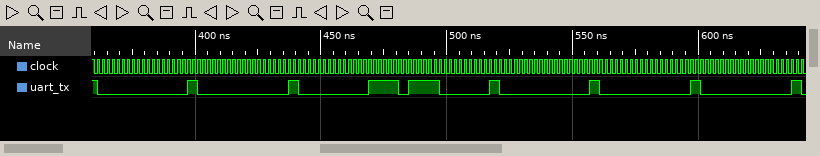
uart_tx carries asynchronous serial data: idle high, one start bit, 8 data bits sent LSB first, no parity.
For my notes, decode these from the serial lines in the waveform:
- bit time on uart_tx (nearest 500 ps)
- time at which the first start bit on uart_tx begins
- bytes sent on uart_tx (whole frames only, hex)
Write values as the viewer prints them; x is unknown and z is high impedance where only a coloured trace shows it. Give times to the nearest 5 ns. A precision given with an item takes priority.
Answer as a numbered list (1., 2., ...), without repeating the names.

1. 4000 ps
2. 360 ns
3. 00, 00, C0, 07, 00, 00, 00
